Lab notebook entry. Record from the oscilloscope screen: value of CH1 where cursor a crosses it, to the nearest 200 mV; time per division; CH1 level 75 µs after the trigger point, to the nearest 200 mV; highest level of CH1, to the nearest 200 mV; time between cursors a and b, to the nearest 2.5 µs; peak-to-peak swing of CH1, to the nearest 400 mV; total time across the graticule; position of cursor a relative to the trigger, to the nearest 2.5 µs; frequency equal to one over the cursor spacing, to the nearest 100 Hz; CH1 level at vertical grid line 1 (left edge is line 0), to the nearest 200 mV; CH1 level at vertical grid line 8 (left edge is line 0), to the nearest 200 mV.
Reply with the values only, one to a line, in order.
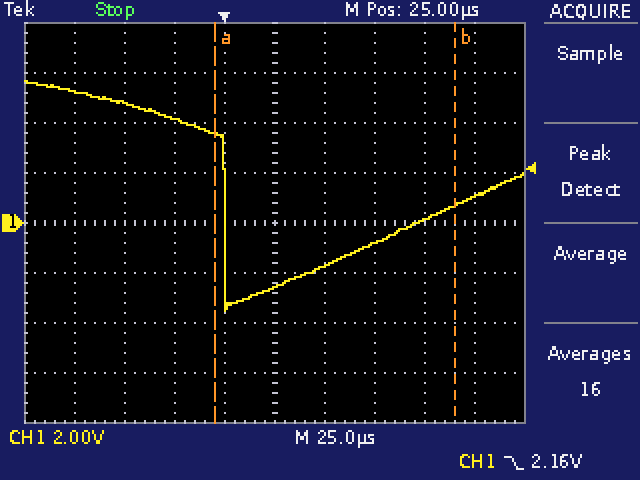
3.6 V
25 µs
-800 mV
5.6 V
120.0 µs
9.2 V
250 µs
-5.0 µs
8.3 kHz
5.2 V
200 mV
